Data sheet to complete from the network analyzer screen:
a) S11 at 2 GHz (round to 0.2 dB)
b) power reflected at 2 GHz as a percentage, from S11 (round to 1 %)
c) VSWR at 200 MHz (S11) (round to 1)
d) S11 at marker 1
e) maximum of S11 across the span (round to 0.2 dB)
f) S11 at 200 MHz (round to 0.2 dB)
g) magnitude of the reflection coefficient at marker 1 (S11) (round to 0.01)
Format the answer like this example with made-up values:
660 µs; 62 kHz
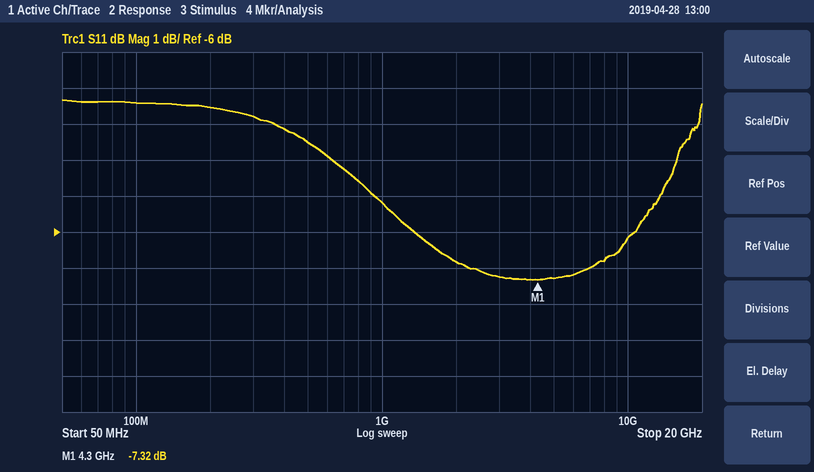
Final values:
-6.8 dB; 21 %; 7; -7.32 dB; -2.4 dB; -2.6 dB; 0.43
